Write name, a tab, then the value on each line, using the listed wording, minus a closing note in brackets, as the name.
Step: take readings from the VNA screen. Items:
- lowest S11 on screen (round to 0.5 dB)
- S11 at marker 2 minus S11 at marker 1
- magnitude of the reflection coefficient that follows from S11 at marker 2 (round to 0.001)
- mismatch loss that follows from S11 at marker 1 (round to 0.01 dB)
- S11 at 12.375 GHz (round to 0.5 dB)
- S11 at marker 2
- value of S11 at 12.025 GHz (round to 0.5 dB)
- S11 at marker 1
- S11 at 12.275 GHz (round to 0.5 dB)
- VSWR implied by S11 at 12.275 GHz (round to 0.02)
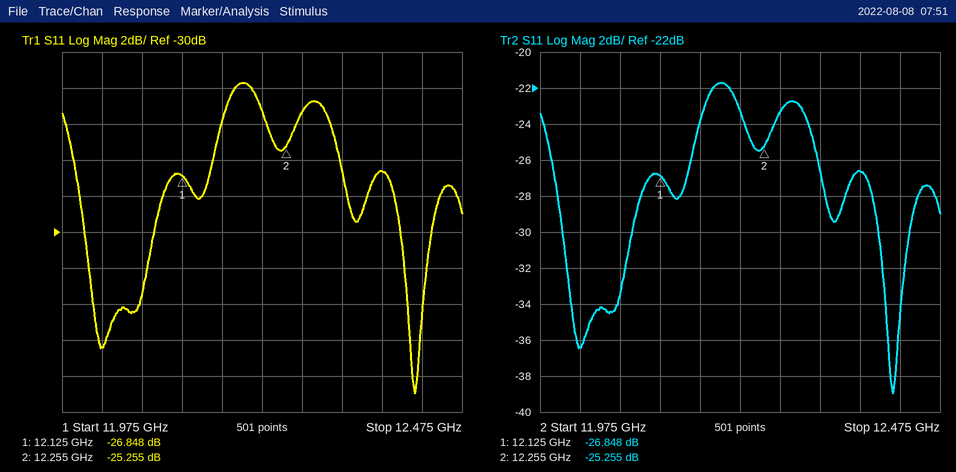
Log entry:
lowest S11 on screen	-39.0 dB
S11 at marker 2 minus S11 at marker 1	1.593 dB
magnitude of the reflection coefficient that follows from S11 at marker 2	0.055
mismatch loss that follows from S11 at marker 1	0.01 dB
S11 at 12.375 GHz	-26.5 dB
S11 at marker 2	-25.255 dB
value of S11 at 12.025 GHz	-36.5 dB
S11 at marker 1	-26.848 dB
S11 at 12.275 GHz	-23.5 dB
VSWR implied by S11 at 12.275 GHz	1.14
